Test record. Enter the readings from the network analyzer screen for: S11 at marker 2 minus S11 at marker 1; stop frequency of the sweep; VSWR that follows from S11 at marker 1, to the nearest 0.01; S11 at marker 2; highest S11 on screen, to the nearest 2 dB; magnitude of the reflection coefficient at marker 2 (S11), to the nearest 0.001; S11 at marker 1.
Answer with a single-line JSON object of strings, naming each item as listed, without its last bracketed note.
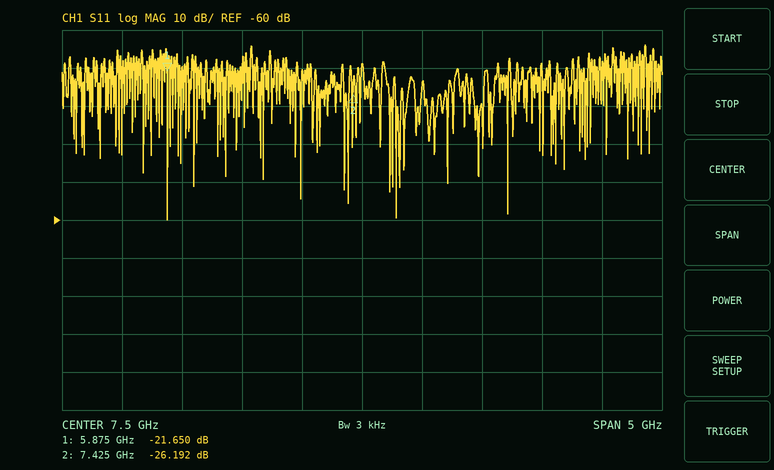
{"S11 at marker 2 minus S11 at marker 1": "-4.542 dB", "stop frequency of the sweep": "10 GHz", "VSWR that follows from S11 at marker 1, to the nearest 0.01": "1.18", "S11 at marker 2": "-26.192 dB", "highest S11 on screen, to the nearest 2 dB": "-14 dB", "magnitude of the reflection coefficient at marker 2 (S11), to the nearest 0.001": "0.049", "S11 at marker 1": "-21.650 dB"}
